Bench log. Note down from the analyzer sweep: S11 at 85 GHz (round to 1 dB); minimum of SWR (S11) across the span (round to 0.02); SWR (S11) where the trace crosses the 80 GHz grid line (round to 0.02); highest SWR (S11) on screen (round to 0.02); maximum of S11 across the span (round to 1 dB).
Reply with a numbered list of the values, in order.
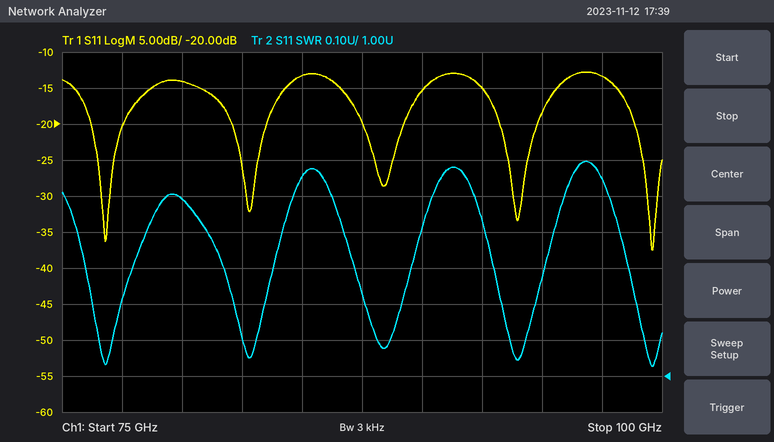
1. -13 dB
2. 1.02
3. 1.50
4. 1.60
5. -13 dB
